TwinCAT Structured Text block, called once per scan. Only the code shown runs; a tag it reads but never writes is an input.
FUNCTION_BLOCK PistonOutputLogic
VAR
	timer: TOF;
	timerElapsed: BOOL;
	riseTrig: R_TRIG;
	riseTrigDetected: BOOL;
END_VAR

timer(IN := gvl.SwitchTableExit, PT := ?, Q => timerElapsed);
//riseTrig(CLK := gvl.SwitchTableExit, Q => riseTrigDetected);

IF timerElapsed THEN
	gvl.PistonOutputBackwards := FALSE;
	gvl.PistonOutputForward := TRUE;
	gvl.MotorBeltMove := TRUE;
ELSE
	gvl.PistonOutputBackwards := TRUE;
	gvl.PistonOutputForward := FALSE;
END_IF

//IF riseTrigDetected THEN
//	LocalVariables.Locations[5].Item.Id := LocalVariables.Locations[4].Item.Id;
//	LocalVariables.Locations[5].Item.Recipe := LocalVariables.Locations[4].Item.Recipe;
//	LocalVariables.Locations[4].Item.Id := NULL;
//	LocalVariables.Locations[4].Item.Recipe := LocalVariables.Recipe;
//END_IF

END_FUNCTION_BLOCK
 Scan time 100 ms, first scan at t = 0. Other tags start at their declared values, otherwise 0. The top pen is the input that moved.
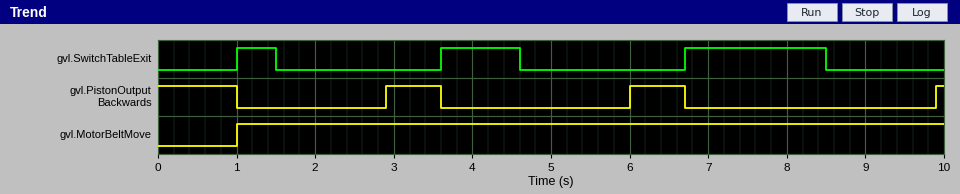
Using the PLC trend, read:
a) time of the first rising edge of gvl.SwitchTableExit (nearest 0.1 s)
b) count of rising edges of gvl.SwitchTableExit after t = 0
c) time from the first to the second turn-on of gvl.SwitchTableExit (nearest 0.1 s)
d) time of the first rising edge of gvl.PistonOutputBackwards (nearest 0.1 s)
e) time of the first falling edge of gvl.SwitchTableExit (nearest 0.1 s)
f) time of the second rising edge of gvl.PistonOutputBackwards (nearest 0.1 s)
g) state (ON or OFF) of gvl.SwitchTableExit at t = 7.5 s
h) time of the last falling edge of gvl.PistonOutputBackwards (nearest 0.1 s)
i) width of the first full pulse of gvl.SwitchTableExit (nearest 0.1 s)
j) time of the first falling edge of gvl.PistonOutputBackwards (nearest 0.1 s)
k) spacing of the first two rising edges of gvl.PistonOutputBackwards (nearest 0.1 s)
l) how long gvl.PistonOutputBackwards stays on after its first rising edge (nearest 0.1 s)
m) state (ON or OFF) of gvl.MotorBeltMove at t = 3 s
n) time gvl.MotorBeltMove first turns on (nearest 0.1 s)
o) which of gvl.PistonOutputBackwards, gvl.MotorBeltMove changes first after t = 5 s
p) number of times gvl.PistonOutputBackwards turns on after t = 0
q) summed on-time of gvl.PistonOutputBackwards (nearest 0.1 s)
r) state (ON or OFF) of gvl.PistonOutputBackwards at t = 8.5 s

1.0 s
3
2.6 s
2.9 s
1.5 s
6.0 s
ON
6.7 s
0.5 s
1.0 s
3.1 s
0.7 s
ON
1.0 s
gvl.PistonOutputBackwards
3
2.5 s
OFF
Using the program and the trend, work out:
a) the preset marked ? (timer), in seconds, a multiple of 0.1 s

1.4 s
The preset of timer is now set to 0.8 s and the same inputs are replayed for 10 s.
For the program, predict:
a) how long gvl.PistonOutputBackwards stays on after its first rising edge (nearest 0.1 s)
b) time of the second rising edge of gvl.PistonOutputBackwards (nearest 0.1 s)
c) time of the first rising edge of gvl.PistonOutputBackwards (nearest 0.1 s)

1.3 s
5.4 s
2.3 s
